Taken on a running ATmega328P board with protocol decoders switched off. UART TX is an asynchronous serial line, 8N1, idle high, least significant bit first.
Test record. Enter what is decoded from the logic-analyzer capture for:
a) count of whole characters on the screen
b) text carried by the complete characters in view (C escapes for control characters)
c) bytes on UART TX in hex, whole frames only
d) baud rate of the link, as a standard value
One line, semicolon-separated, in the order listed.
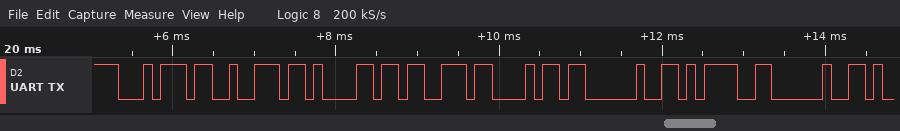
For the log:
8; "trash = "; 0x74 0x72 0x61 0x73 0x68 0x20 0x3D 0x20; 9600 baud
